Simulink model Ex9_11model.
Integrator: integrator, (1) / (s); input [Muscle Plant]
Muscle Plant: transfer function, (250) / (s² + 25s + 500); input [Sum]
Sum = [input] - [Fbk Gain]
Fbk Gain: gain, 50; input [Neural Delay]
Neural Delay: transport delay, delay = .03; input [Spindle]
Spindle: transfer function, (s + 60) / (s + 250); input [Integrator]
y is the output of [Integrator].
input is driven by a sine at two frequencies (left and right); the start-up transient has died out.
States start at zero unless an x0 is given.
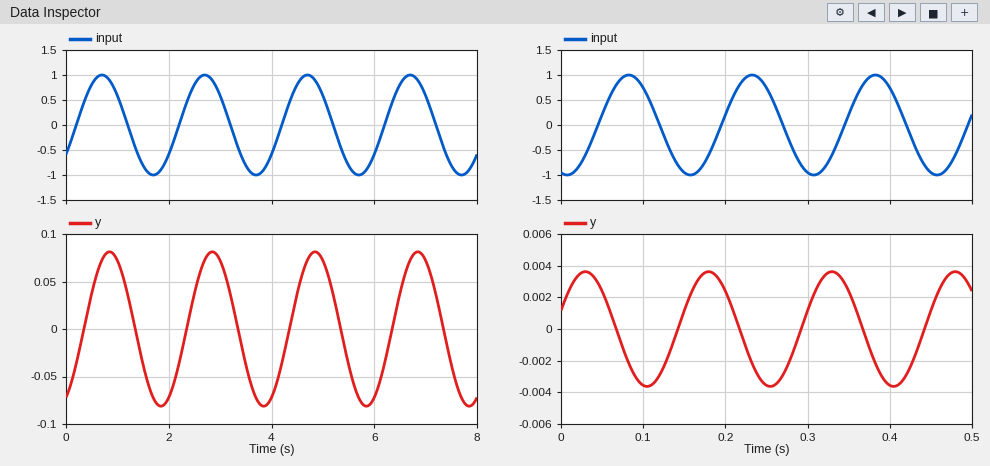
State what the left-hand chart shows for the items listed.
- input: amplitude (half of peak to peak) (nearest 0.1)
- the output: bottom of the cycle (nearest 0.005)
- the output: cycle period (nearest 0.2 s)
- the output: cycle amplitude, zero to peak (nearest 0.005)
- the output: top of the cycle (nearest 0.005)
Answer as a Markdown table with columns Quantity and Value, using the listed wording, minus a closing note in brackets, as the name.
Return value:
| Quantity | Value |
|---|---|
| input: amplitude (half of peak to peak) | 1.0 |
| the output: bottom of the cycle | -0.080 |
| the output: cycle period | 2.0 s |
| the output: cycle amplitude, zero to peak | 0.080 |
| the output: top of the cycle | 0.080 |
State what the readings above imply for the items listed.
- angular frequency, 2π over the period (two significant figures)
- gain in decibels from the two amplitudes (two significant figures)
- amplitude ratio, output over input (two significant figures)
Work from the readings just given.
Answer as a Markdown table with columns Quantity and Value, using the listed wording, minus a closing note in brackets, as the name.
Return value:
| Quantity | Value |
|---|---|
| angular frequency, 2π over the period | 3.1 rad/s |
| gain in decibels from the two amplitudes | -22 dB |
| amplitude ratio, output over input | 0.080 |
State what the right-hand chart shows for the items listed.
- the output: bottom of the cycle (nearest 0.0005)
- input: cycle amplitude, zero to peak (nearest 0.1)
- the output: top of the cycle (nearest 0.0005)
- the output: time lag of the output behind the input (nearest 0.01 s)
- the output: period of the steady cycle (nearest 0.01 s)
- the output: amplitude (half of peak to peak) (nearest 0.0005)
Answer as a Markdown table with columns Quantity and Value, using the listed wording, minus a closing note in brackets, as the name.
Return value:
| Quantity | Value |
|---|---|
| the output: bottom of the cycle | -0.0035 |
| input: cycle amplitude, zero to peak | 1.0 |
| the output: top of the cycle | 0.0035 |
| the output: time lag of the output behind the input | 0.10 s |
| the output: period of the steady cycle | 0.15 s |
| the output: amplitude (half of peak to peak) | 0.0035 |
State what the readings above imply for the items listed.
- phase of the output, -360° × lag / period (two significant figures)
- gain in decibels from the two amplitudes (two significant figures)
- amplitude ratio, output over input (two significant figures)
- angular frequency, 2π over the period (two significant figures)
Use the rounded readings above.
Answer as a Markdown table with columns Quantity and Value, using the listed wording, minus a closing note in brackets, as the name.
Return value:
| Quantity | Value |
|---|---|
| phase of the output, -360° × lag / period | -240° |
| gain in decibels from the two amplitudes | -49 dB |
| amplitude ratio, output over input | 0.0035 |
| angular frequency, 2π over the period | 42 rad/s |
